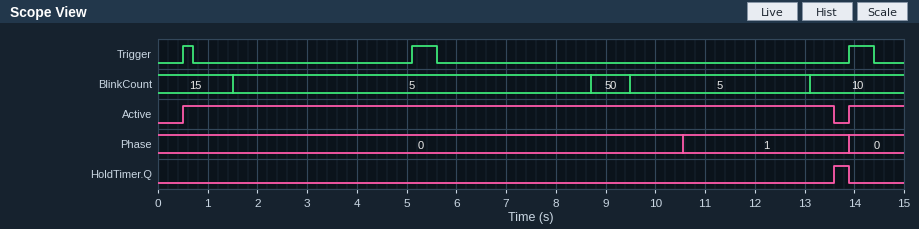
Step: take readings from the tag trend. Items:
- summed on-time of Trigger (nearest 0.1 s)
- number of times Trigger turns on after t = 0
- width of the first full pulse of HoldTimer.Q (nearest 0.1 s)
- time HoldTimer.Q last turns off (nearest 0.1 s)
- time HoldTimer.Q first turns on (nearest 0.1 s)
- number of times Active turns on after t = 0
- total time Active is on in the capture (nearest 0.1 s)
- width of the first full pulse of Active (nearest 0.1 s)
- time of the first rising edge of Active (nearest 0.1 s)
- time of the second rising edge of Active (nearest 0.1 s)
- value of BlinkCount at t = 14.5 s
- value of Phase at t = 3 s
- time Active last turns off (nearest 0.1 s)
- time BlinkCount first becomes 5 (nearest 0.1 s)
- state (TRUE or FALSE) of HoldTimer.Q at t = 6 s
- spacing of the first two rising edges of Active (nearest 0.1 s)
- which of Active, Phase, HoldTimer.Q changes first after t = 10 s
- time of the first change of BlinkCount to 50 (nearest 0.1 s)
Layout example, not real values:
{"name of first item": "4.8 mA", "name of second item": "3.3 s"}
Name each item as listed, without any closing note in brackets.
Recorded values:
{"summed on-time of Trigger": "1.2 s", "number of times Trigger turns on after t = 0": "3", "width of the first full pulse of HoldTimer.Q": "0.3 s", "time HoldTimer.Q last turns off": "13.9 s", "time HoldTimer.Q first turns on": "13.6 s", "number of times Active turns on after t = 0": "2", "total time Active is on in the capture": "14.2 s", "width of the first full pulse of Active": "13.1 s", "time of the first rising edge of Active": "0.5 s", "time of the second rising edge of Active": "13.9 s", "value of BlinkCount at t = 14.5 s": "10", "value of Phase at t = 3 s": "0", "time Active last turns off": "13.6 s", "time BlinkCount first becomes 5": "1.5 s", "state (TRUE or FALSE) of HoldTimer.Q at t = 6 s": "FALSE", "spacing of the first two rising edges of Active": "13.4 s", "which of Active, Phase, HoldTimer.Q changes first after t = 10 s": "Phase", "time of the first change of BlinkCount to 50": "8.7 s"}
